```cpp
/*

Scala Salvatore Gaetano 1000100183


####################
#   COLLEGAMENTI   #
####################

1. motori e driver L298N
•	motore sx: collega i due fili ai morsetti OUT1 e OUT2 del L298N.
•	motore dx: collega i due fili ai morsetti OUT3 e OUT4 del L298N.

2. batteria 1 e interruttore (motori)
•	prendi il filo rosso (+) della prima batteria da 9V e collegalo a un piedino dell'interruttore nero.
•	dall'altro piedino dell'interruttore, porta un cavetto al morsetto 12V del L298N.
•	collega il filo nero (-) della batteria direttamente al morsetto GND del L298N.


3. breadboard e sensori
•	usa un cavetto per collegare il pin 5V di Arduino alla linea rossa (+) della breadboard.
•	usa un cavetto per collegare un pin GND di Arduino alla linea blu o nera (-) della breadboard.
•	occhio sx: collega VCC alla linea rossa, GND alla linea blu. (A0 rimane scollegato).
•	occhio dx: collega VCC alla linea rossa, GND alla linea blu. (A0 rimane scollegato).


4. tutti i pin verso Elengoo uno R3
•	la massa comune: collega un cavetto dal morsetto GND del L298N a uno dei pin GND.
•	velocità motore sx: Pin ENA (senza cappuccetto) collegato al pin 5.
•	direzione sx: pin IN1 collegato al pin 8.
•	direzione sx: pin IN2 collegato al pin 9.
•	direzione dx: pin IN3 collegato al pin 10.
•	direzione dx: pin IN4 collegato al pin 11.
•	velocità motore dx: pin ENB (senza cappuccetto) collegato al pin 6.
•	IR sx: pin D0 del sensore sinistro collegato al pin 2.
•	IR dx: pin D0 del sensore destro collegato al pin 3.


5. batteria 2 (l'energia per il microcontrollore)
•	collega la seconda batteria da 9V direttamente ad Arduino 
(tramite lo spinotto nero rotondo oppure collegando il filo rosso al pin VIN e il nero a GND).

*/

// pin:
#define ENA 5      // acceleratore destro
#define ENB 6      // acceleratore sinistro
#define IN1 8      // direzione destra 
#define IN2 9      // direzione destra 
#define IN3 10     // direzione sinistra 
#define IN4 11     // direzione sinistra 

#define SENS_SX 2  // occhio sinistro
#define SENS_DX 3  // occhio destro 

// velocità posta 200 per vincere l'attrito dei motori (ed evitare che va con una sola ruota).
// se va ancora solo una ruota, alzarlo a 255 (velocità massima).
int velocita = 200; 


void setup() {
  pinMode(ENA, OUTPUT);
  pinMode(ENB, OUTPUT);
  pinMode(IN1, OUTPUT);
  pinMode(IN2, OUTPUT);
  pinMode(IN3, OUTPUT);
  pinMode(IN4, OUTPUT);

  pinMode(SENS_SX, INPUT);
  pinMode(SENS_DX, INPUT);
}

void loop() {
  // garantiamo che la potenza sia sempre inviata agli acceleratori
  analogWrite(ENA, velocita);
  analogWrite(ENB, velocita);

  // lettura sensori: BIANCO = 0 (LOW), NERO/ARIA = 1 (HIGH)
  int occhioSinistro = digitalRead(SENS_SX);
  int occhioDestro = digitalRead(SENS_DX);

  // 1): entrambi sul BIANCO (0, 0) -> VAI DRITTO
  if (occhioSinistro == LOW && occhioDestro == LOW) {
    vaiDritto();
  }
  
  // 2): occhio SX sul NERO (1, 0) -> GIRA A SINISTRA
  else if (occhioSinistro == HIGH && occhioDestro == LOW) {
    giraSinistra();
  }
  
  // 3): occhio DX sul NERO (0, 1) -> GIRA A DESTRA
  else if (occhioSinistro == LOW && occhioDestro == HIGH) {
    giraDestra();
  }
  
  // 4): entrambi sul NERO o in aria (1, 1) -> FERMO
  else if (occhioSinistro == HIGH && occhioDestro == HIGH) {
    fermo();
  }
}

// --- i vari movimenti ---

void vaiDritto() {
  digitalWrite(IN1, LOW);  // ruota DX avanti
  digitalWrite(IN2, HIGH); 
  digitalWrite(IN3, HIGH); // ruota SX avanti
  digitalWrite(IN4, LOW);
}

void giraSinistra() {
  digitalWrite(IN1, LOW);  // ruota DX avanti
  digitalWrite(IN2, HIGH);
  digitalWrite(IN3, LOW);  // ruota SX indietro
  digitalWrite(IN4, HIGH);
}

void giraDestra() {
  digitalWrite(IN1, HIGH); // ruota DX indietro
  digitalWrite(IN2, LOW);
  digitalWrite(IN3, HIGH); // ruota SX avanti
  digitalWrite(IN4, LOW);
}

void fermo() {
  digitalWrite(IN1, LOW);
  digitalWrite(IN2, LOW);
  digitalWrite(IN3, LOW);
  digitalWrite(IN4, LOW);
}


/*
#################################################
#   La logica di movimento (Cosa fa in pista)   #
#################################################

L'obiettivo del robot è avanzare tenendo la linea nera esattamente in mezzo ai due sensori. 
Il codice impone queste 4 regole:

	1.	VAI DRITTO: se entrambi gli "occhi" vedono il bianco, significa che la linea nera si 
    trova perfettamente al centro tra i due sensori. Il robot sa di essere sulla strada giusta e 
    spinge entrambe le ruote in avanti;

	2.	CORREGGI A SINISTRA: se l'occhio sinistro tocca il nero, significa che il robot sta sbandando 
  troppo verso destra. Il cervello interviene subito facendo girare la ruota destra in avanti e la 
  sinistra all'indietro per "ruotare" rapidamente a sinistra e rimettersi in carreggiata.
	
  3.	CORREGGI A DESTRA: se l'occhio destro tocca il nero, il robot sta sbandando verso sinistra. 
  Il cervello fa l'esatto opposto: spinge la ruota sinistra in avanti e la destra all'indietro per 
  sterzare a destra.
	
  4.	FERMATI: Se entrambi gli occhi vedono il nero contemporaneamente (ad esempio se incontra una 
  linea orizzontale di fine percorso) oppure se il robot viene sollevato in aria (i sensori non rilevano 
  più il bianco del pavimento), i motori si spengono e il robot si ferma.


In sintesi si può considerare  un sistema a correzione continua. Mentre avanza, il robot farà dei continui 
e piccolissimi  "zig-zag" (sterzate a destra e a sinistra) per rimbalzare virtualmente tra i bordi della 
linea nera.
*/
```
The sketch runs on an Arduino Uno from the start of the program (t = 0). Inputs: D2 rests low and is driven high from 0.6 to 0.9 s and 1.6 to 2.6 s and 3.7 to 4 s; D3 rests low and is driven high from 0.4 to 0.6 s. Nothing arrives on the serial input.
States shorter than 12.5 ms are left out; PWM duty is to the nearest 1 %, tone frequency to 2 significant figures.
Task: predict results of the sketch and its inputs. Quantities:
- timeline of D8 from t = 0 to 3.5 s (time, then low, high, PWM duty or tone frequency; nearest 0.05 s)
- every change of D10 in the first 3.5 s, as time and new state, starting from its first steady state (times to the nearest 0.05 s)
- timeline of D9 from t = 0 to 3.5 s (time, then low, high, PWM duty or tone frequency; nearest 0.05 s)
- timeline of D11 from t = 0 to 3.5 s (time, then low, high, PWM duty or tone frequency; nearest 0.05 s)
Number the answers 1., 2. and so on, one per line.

1. 0 s low; 0.4 s high; 0.6 s low
2. 0 s high; 0.6 s low; 0.9 s high; 1.6 s low; 2.6 s high
3. 0 s high; 0.4 s low; 0.6 s high
4. 0 s low; 0.6 s high; 0.9 s low; 1.6 s high; 2.6 s low
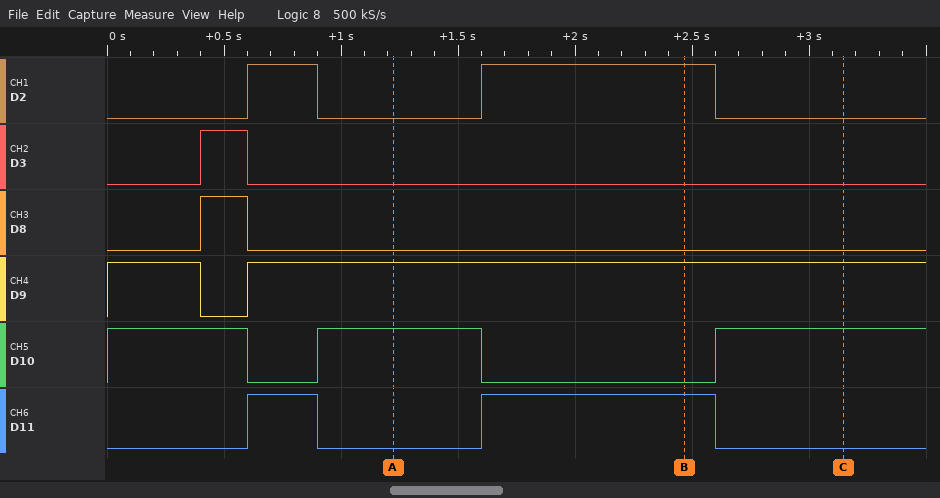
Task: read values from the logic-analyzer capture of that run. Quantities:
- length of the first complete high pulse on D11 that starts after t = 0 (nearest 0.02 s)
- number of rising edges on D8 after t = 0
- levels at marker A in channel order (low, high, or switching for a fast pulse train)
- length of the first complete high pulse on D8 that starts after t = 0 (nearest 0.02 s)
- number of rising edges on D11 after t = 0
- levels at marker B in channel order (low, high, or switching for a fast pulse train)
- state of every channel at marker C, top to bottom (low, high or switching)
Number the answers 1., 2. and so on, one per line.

1. 0.30 s
2. 1
3. D2 low, D3 low, D8 low, D9 high, D10 high, D11 low
4. 0.20 s
5. 2
6. D2 high, D3 low, D8 low, D9 high, D10 low, D11 high
7. D2 low, D3 low, D8 low, D9 high, D10 high, D11 low
